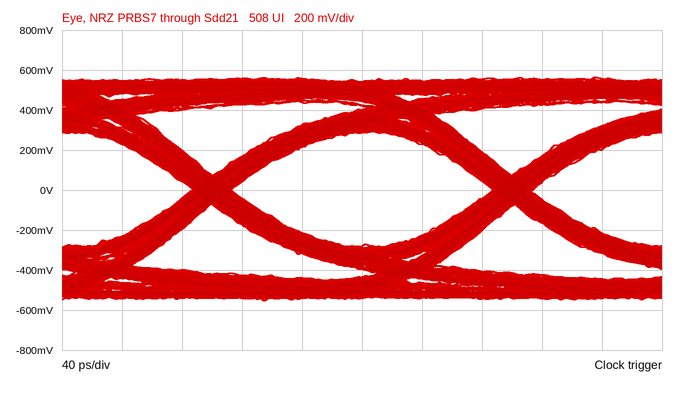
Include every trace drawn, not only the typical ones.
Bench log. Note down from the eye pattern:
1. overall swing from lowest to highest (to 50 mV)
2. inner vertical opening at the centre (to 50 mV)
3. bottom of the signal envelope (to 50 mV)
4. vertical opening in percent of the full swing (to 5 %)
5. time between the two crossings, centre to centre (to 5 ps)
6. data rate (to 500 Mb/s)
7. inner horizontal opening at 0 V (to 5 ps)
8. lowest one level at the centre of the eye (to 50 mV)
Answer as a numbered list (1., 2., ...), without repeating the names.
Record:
1. 1.10 V
2. 550 mV
3. -550 mV
4. 50 %
5. 200 ps
6. 5.0 Gb/s
7. 175 ps
8. 300 mV
